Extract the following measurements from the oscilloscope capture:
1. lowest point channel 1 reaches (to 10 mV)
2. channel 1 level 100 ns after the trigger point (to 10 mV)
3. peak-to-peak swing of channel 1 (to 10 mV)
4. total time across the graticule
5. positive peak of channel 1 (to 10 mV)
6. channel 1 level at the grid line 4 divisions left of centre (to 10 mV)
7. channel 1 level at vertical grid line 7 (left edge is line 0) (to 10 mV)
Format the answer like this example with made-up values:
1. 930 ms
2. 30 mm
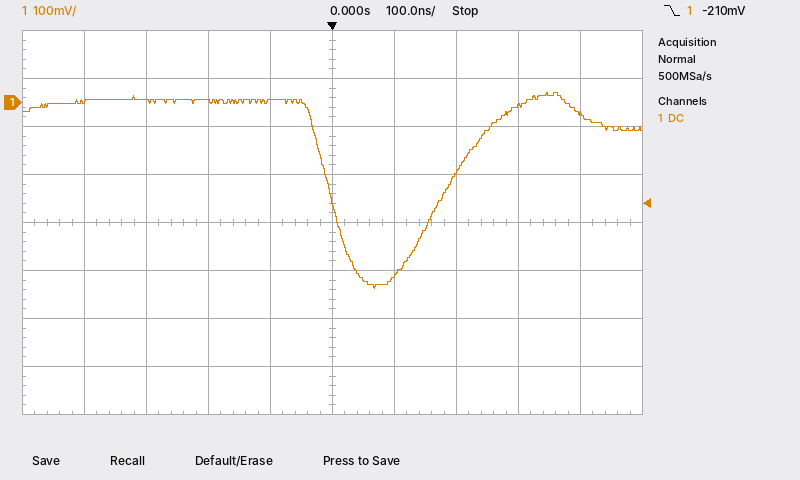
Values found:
1. -390 mV
2. -360 mV
3. 410 mV
4. 1 µs
5. 20 mV
6. 0 mV
7. -150 mV
